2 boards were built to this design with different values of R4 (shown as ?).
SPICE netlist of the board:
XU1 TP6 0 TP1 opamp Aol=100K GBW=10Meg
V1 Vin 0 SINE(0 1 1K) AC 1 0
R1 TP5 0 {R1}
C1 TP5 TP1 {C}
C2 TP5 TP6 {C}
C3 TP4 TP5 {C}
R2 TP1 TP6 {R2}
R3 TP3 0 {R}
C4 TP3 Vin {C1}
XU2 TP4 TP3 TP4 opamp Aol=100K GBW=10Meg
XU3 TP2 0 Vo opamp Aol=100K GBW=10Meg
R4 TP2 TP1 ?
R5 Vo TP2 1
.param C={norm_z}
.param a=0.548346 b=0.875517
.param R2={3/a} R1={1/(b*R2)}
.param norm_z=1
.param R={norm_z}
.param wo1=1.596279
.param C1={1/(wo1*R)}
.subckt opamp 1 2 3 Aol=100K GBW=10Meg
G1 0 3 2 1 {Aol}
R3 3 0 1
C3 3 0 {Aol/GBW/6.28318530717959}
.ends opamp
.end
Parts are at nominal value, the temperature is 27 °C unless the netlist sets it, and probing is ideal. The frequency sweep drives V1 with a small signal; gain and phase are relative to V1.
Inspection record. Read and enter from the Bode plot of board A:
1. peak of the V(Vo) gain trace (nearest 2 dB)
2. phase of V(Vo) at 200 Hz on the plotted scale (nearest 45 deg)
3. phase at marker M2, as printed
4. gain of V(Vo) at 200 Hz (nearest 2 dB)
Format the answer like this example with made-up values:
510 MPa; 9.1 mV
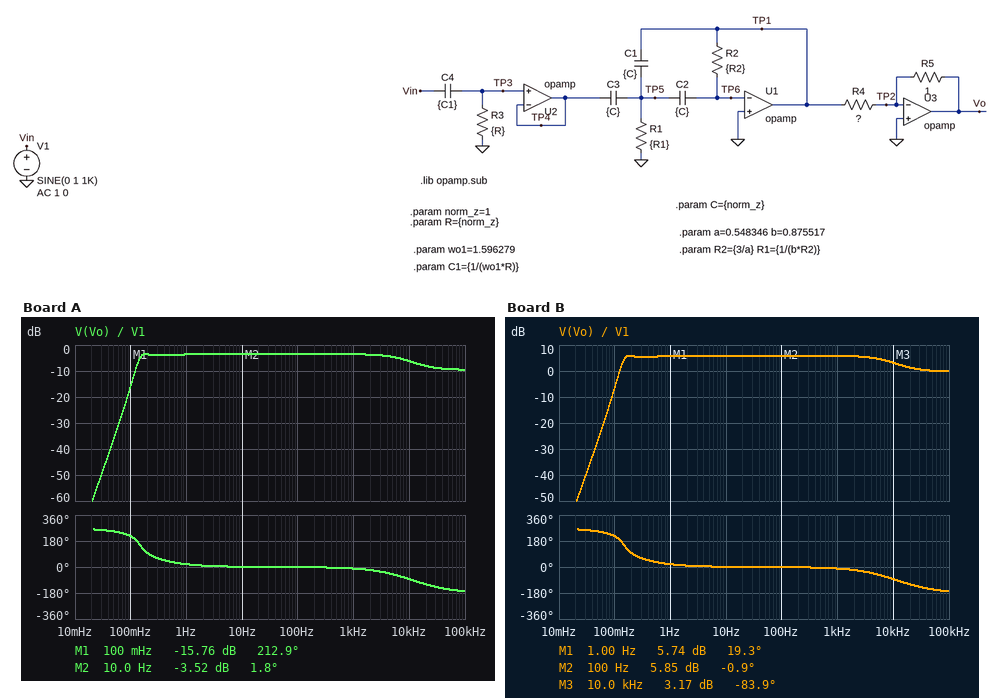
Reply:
-4 dB; 0 deg; 1.8 deg; -4 dB
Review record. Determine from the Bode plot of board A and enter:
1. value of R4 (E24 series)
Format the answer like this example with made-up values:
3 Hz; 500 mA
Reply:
1.5 Ω
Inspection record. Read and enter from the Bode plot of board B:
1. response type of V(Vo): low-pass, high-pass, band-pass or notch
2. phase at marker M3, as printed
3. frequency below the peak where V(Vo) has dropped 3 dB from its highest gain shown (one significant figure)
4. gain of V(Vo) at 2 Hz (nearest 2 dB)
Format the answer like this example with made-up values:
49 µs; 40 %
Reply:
high-pass; -83.9 deg; 100 mHz; 6 dB
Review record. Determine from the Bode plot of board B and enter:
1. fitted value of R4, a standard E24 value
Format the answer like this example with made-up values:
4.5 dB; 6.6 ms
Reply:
0.51 Ω
